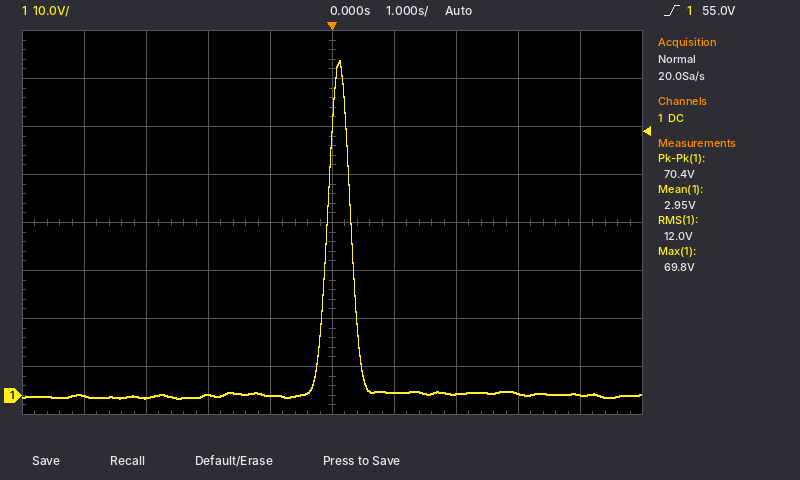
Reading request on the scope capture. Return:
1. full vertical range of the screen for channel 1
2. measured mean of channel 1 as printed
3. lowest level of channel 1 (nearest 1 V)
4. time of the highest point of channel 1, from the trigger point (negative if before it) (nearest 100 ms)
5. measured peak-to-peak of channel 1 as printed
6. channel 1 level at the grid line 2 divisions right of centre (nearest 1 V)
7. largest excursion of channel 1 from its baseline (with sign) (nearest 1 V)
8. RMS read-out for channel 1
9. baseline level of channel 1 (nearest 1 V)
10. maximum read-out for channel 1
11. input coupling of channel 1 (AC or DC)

80 V
2.95 V
-1 V
+100 ms
70.4 V
0 V
+70 V
12.0 V
0 V
69.8 V
DC
